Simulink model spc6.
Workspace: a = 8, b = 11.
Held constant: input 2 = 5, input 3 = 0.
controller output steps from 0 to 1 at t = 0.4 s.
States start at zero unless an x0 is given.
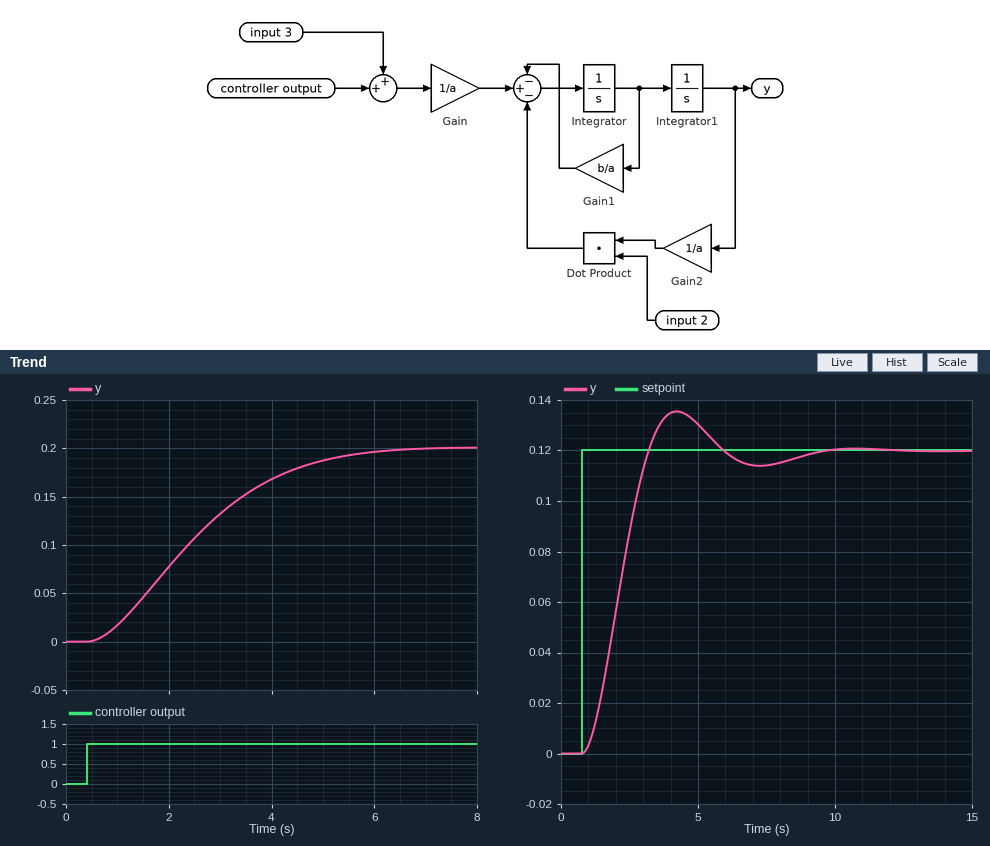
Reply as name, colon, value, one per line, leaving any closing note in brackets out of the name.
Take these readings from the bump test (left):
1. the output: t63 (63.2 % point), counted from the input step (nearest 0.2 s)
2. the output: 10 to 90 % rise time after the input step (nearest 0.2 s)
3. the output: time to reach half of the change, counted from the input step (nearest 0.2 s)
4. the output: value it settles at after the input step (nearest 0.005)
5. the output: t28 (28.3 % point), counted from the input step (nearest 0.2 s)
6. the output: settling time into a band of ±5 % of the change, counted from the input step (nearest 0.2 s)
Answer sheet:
the output: t63 (63.2 % point), counted from the input step: 2.4 s
the output: 10 to 90 % rise time after the input step: 3.4 s
the output: time to reach half of the change, counted from the input step: 2.0 s
the output: value it settles at after the input step: 0.200
the output: t28 (28.3 % point), counted from the input step: 1.2 s
the output: settling time into a band of ±5 % of the change, counted from the input step: 4.8 s
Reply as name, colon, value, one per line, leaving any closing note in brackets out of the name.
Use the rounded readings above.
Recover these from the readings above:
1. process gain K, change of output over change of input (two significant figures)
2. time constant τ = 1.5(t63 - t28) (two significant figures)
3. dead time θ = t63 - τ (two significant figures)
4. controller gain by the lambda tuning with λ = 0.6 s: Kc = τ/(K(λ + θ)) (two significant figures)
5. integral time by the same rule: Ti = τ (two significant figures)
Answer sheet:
process gain K, change of output over change of input: 0.20
time constant τ = 1.5(t63 - t28): 1.8 s
dead time θ = t63 - τ: 0.60 s
controller gain by the lambda tuning with λ = 0.6 s: Kc = τ/(K(λ + θ)): 7.5
integral time by the same rule: Ti = τ: 1.8 s
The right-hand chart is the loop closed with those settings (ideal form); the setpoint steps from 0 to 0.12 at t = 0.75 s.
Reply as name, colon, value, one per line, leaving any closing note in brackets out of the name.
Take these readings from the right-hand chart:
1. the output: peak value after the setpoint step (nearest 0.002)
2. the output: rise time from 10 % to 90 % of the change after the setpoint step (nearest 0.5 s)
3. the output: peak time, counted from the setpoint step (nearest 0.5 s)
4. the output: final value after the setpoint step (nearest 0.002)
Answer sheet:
the output: peak value after the setpoint step: 0.136
the output: rise time from 10 % to 90 % of the change after the setpoint step: 1.5 s
the output: peak time, counted from the setpoint step: 3.5 s
the output: final value after the setpoint step: 0.120
